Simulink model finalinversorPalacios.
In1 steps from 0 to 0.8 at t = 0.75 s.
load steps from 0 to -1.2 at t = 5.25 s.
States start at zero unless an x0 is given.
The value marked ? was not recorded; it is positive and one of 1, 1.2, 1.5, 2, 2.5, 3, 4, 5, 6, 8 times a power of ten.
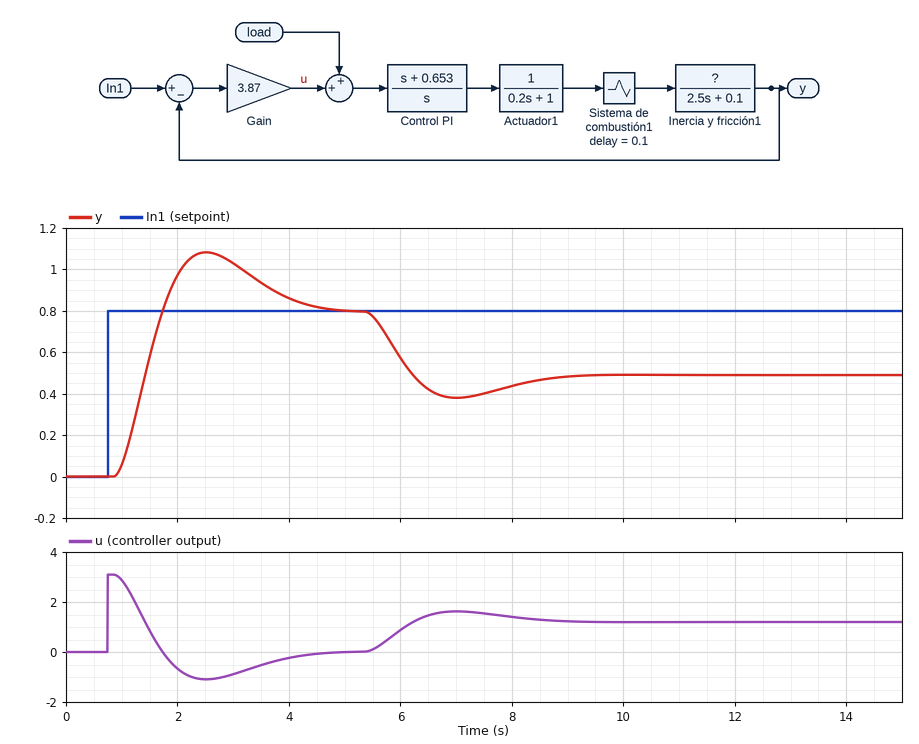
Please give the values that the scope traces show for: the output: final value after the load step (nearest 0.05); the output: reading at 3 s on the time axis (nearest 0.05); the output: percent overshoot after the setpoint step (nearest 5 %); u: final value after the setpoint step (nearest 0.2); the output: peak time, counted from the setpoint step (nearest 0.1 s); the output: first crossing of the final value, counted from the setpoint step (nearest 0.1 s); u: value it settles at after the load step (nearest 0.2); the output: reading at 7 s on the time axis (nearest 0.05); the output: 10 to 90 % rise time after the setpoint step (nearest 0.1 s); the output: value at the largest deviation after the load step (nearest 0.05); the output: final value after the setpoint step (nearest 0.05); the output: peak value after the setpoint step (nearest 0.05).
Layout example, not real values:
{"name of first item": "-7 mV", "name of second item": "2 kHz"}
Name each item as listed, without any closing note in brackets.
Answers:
{"the output: final value after the load step": "0.50", "the output: reading at 3 s on the time axis": "1.05", "the output: percent overshoot after the setpoint step": "35 %", "u: final value after the setpoint step": "0.0", "the output: peak time, counted from the setpoint step": "1.8 s", "the output: first crossing of the final value, counted from the setpoint step": "1.0 s", "u: value it settles at after the load step": "1.2", "the output: reading at 7 s on the time axis": "0.40", "the output: 10 to 90 % rise time after the setpoint step": "0.6 s", "the output: value at the largest deviation after the load step": "0.40", "the output: final value after the setpoint step": "0.80", "the output: peak value after the setpoint step": "1.10"}
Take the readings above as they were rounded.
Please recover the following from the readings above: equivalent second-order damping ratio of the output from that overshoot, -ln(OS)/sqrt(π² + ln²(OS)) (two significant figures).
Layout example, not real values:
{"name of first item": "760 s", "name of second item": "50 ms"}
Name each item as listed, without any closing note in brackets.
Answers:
{"equivalent second-order damping ratio of the output from that overshoot, -ln(OS)/sqrt(π² + ln²(OS))": "0.32"}
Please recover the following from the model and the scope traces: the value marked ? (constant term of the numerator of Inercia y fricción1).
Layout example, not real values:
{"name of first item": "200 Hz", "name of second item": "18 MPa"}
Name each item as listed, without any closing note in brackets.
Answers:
{"the value marked ?": "1"}
